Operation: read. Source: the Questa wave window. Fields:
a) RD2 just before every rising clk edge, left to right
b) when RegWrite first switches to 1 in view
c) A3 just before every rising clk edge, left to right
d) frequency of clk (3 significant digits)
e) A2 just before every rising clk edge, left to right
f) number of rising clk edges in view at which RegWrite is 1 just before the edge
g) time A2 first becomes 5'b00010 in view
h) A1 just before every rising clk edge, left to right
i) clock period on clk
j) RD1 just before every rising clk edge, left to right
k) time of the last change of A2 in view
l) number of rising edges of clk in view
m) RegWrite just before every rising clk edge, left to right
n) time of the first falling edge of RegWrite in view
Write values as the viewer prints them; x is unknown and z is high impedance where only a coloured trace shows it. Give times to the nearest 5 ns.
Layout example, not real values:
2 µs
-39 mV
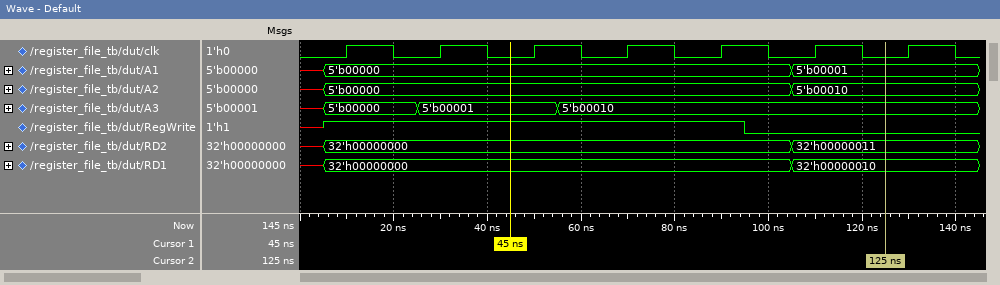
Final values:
32'h00000000, 32'h00000000, 32'h00000000, 32'h00000000, 32'h00000000, 32'h00000011, 32'h00000011
5 ns
5'b00000, 5'b00001, 5'b00001, 5'b00010, 5'b00010, 5'b00010, 5'b00010
50.0 MHz
5'b00000, 5'b00000, 5'b00000, 5'b00000, 5'b00000, 5'b00010, 5'b00010
5
105 ns
5'b00000, 5'b00000, 5'b00000, 5'b00000, 5'b00000, 5'b00001, 5'b00001
20 ns
32'h00000000, 32'h00000000, 32'h00000000, 32'h00000000, 32'h00000000, 32'h00000010, 32'h00000010
105 ns
7
1 1 1 1 1 0 0
95 ns
